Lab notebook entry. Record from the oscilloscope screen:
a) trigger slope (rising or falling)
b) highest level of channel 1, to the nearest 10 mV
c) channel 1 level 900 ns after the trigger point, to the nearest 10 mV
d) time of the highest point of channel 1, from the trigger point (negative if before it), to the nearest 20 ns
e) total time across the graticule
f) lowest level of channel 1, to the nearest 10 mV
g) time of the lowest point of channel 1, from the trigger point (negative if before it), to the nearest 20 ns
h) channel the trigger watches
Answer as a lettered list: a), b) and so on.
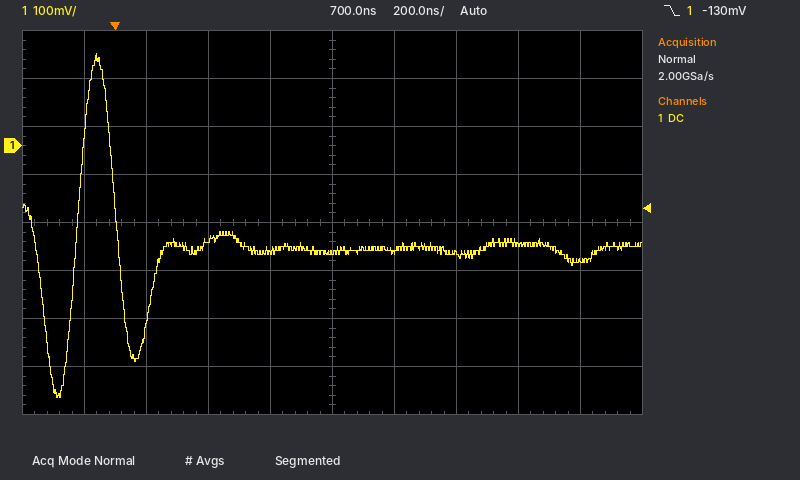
a) falling
b) 190 mV
c) -220 mV
d) -60 ns
e) 2 µs
f) -520 mV
g) -180 ns
h) channel 1
